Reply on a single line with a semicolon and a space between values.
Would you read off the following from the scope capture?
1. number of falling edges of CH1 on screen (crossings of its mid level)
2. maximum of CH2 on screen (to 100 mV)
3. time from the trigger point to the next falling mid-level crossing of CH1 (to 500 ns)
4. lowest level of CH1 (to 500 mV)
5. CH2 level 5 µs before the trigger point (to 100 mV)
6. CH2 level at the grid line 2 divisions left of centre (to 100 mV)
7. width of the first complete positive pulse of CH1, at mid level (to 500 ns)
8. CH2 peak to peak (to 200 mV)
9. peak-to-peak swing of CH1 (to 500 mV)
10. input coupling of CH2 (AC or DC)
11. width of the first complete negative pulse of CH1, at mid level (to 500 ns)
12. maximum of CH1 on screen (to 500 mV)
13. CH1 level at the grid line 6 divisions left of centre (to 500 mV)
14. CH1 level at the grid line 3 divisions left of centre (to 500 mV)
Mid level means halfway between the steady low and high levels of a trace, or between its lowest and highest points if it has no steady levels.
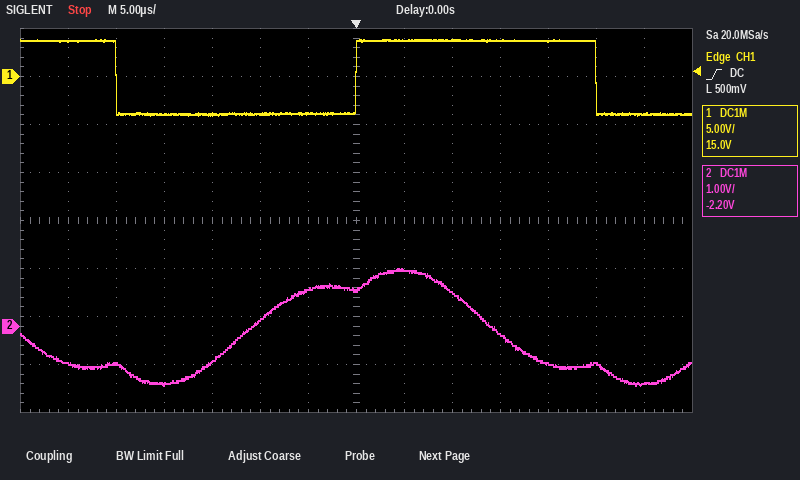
2; 1.2 V; 25.0 µs; -4.0 V; 800 mV; 100 mV; 25.0 µs; 2.4 V; 8.0 V; DC; 25.0 µs; 4.0 V; 3.5 V; -4.0 V
